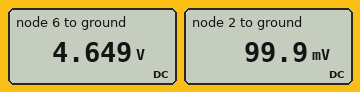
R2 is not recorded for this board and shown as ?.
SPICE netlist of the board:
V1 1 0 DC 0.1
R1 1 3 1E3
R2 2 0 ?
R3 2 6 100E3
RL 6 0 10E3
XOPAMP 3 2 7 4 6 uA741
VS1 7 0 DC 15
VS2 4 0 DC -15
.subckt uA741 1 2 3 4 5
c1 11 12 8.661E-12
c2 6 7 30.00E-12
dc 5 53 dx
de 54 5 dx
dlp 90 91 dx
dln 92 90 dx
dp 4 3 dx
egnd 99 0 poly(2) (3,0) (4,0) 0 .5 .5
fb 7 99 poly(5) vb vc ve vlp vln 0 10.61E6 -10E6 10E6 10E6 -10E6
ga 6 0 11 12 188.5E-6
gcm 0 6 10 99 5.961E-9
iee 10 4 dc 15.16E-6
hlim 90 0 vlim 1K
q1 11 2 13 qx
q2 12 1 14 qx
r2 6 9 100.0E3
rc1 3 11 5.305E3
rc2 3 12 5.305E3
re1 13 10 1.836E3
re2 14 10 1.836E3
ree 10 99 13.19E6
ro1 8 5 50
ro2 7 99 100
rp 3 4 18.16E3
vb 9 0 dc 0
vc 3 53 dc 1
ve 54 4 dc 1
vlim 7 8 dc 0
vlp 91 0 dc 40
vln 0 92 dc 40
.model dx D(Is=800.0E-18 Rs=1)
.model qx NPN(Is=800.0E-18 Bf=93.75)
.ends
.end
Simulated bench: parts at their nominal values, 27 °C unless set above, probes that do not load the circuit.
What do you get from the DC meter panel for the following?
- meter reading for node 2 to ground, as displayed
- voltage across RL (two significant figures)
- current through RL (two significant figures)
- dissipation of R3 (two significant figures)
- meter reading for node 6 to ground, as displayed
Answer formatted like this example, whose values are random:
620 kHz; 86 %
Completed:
99.9 mV; 4.6 V; 460 µA; 210 µW; 4.649 V
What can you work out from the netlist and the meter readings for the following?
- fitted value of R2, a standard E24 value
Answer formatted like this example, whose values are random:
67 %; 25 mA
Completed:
2.2 kΩ
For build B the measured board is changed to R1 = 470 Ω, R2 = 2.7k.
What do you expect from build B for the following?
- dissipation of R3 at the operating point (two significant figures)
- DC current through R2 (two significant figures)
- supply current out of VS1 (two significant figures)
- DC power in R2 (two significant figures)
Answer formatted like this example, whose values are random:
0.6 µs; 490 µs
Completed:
140 µW; 37 µA; 1.7 mA; 3.7 µW
